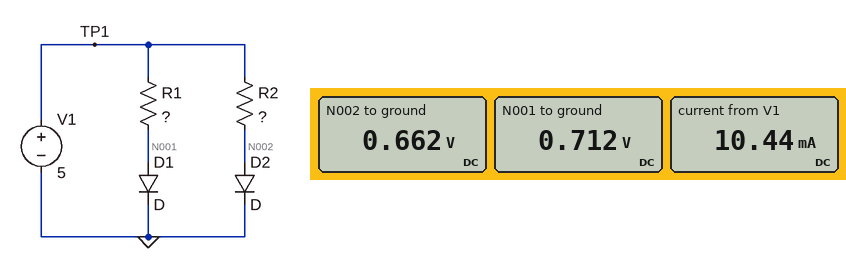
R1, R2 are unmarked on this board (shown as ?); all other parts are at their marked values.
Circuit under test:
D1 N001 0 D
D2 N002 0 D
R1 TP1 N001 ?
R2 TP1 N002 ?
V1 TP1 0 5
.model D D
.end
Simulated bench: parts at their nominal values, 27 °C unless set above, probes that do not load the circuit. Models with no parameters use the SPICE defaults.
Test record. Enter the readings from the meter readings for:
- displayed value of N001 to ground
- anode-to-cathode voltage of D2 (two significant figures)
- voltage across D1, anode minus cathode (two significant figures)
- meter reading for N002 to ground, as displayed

0.712 V
660 mV
710 mV
0.662 V
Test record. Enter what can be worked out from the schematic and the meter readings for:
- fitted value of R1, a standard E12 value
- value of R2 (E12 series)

470 Ω
3.3 kΩ
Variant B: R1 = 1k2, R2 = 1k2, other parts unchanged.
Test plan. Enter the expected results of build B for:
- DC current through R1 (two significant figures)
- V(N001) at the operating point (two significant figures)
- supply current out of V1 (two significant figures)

3.6 mA
690 mV
7.2 mA
